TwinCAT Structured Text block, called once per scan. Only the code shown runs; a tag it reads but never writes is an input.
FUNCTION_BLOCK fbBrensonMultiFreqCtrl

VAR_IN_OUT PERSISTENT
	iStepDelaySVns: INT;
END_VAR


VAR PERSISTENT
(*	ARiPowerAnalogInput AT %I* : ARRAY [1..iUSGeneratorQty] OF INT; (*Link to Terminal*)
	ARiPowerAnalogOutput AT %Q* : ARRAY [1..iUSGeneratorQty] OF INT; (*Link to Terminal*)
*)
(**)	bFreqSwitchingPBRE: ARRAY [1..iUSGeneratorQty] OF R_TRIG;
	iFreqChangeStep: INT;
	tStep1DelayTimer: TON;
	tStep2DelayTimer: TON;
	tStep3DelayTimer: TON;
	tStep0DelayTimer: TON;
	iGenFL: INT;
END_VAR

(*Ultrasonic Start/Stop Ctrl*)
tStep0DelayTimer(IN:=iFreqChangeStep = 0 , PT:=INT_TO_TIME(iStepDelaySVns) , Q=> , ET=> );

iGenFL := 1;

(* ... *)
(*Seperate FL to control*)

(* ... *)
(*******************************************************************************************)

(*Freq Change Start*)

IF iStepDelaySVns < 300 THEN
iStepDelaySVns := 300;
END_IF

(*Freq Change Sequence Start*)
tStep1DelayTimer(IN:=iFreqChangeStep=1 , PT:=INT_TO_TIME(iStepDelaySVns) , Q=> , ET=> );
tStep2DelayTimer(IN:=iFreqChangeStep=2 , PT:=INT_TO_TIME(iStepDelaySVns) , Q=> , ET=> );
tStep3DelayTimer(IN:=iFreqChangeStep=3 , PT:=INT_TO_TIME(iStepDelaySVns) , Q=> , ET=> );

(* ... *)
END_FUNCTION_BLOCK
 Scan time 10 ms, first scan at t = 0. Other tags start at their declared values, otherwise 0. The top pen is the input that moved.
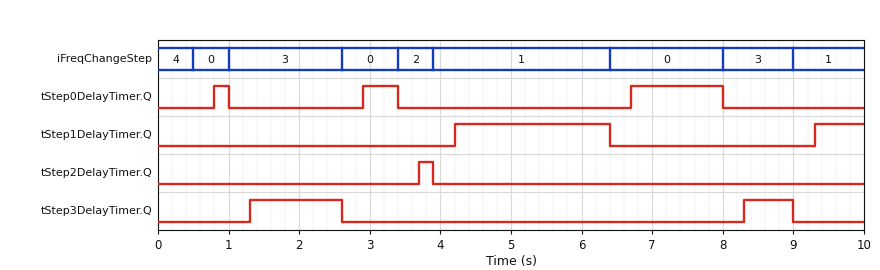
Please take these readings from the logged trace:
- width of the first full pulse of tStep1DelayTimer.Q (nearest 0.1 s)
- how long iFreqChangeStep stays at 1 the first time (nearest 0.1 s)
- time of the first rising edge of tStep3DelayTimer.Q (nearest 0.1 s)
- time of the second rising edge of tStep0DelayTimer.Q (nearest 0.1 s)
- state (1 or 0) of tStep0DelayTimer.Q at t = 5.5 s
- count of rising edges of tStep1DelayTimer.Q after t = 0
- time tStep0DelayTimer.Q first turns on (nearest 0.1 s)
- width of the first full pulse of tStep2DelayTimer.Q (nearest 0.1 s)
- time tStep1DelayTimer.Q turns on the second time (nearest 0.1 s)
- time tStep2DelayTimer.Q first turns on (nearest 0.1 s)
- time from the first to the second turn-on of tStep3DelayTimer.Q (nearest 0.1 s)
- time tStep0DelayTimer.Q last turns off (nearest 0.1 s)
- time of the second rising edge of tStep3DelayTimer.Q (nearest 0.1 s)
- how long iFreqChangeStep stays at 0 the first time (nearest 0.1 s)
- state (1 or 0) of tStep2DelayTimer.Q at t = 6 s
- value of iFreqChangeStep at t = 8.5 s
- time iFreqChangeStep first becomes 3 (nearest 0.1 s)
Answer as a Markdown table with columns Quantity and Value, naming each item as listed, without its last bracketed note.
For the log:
| Quantity | Value |
|---|---|
| width of the first full pulse of tStep1DelayTimer.Q | 2.2 s |
| how long iFreqChangeStep stays at 1 the first time | 2.5 s |
| time of the first rising edge of tStep3DelayTimer.Q | 1.3 s |
| time of the second rising edge of tStep0DelayTimer.Q | 2.9 s |
| state (1 or 0) of tStep0DelayTimer.Q at t = 5.5 s | 0 |
| count of rising edges of tStep1DelayTimer.Q after t = 0 | 2 |
| time tStep0DelayTimer.Q first turns on | 0.8 s |
| width of the first full pulse of tStep2DelayTimer.Q | 0.2 s |
| time tStep1DelayTimer.Q turns on the second time | 9.3 s |
| time tStep2DelayTimer.Q first turns on | 3.7 s |
| time from the first to the second turn-on of tStep3DelayTimer.Q | 7.0 s |
| time tStep0DelayTimer.Q last turns off | 8.0 s |
| time of the second rising edge of tStep3DelayTimer.Q | 8.3 s |
| how long iFreqChangeStep stays at 0 the first time | 0.5 s |
| state (1 or 0) of tStep2DelayTimer.Q at t = 6 s | 0 |
| value of iFreqChangeStep at t = 8.5 s | 3 |
| time iFreqChangeStep first becomes 3 | 1.0 s |
